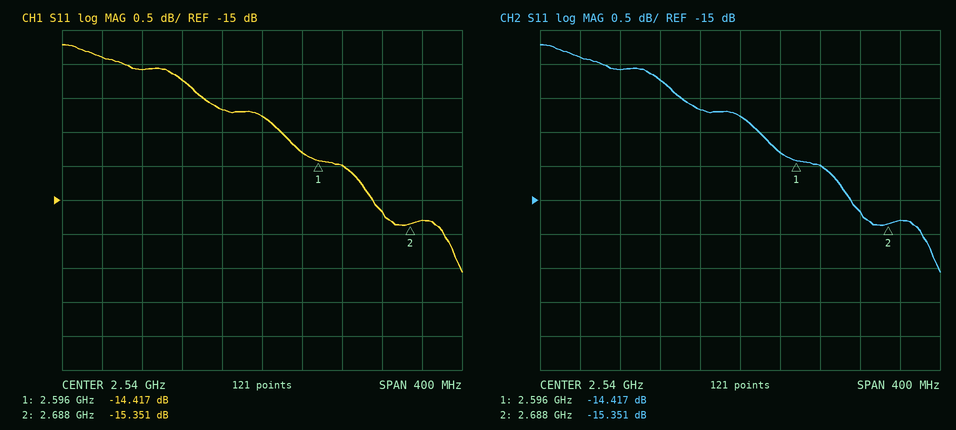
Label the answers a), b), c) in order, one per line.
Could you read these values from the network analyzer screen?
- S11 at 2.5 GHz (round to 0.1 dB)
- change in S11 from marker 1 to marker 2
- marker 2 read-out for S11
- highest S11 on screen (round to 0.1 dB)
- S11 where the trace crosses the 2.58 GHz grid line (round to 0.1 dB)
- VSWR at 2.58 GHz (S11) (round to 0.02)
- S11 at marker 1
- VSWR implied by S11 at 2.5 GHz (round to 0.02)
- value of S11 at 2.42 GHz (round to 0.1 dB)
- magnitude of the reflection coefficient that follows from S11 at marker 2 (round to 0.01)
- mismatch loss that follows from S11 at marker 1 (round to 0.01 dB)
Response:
a) -13.7 dB
b) -0.934 dB
c) -15.351 dB
d) -12.7 dB
e) -14.3 dB
f) 1.48
g) -14.417 dB
h) 1.52
i) -13.1 dB
j) 0.17
k) 0.16 dB
